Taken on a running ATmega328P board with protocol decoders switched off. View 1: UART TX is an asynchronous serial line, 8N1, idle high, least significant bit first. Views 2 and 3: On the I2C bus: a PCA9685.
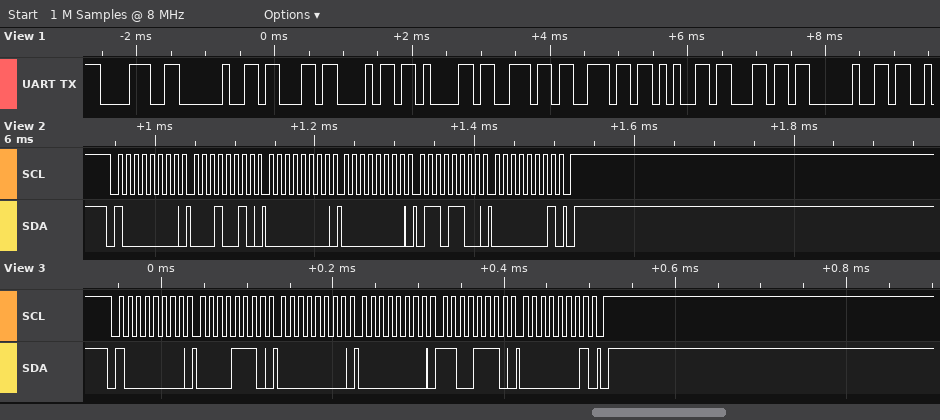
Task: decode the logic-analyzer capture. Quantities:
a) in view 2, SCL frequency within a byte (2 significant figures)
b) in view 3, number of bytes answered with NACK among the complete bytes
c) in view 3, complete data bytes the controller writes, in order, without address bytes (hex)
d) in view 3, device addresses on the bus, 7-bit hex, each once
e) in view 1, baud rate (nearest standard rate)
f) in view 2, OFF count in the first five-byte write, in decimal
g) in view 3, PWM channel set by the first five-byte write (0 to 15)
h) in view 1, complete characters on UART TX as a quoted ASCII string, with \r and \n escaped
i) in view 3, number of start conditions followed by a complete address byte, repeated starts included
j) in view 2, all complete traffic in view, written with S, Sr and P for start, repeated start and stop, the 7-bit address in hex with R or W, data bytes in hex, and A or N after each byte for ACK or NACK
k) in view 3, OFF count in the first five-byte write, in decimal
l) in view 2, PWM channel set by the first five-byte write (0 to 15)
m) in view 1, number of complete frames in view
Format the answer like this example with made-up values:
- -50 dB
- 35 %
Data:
- 100 kHz
- 0
- 0E 00 00 CE 01
- 0x40
- 9600 baud
- 364
- 2
- "8 channel "
- 1
- S 40W A 12 A 00 A 00 A 6C A 01 A P
- 462
- 3
- 10
